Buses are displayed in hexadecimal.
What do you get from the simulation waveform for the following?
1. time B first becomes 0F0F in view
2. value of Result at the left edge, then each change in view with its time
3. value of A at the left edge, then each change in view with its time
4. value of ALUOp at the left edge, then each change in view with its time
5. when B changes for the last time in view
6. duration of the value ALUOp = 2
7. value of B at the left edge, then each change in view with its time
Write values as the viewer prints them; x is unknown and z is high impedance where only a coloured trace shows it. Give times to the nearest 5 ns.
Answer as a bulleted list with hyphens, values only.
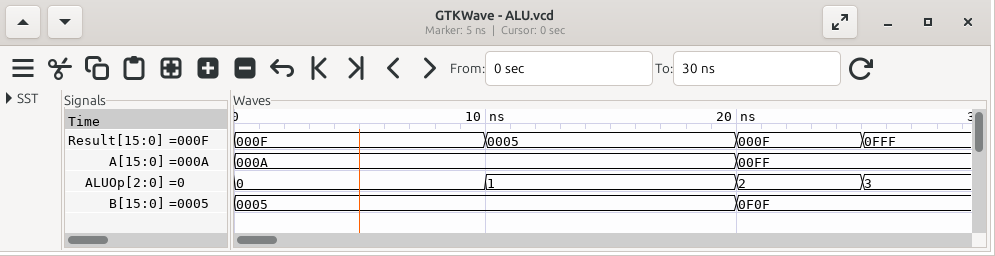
- 20 ns
- 000F, 0005 at 10 ns, 000F at 20 ns, 0FFF at 25 ns
- 000A, 00FF at 20 ns
- 0, 1 at 10 ns, 2 at 20 ns, 3 at 25 ns
- 20 ns
- 5 ns
- 0005, 0F0F at 20 ns
